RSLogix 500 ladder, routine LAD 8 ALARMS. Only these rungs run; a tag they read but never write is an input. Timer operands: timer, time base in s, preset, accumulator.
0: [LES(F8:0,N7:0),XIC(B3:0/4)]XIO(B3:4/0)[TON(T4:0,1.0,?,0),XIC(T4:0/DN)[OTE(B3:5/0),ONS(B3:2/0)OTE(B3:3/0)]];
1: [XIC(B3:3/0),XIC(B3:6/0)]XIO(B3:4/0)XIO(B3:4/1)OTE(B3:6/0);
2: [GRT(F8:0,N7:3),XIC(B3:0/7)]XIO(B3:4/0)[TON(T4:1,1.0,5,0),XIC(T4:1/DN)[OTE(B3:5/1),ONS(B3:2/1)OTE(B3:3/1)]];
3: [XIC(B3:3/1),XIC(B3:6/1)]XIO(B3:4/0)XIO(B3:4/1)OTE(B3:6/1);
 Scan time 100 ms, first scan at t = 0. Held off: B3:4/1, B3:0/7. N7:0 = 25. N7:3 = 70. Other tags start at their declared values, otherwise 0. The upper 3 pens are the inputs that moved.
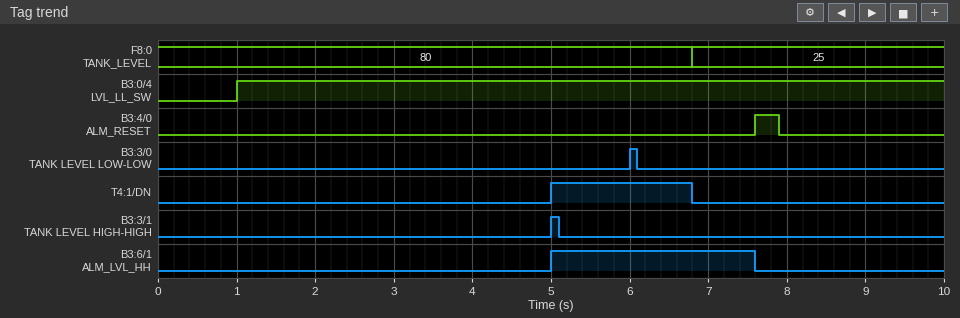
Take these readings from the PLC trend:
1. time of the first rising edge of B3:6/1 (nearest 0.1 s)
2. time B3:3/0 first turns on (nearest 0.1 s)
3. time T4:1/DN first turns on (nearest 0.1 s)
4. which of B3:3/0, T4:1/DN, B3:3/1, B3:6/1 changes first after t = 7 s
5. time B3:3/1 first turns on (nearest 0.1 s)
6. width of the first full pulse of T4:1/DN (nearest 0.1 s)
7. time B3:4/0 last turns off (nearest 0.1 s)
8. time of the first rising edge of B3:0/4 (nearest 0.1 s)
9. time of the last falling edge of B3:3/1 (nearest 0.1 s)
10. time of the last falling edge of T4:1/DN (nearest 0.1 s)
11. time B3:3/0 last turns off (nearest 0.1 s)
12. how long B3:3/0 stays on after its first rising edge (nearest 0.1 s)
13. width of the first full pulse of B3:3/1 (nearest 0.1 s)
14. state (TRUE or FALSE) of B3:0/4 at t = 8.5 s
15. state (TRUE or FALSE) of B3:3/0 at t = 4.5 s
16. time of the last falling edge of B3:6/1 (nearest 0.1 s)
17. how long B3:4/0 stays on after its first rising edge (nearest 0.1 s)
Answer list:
5.0 s
6.0 s
5.0 s
B3:6/1
5.0 s
1.8 s
7.9 s
1.0 s
5.1 s
6.8 s
6.1 s
0.1 s
0.1 s
TRUE
FALSE
7.6 s
0.3 s
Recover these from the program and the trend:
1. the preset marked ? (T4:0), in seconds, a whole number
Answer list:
5 s
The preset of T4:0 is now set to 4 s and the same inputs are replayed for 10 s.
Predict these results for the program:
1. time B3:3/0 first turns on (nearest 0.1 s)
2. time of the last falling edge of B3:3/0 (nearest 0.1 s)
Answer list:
5.0 s
5.1 s
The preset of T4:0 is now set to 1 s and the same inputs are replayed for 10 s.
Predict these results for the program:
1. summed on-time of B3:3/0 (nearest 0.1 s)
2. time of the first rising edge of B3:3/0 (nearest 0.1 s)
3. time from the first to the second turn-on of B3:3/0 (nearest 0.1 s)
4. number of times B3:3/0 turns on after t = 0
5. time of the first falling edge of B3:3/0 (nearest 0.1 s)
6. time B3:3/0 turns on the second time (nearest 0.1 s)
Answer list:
0.2 s
2.0 s
6.9 s
2
2.1 s
8.9 s
